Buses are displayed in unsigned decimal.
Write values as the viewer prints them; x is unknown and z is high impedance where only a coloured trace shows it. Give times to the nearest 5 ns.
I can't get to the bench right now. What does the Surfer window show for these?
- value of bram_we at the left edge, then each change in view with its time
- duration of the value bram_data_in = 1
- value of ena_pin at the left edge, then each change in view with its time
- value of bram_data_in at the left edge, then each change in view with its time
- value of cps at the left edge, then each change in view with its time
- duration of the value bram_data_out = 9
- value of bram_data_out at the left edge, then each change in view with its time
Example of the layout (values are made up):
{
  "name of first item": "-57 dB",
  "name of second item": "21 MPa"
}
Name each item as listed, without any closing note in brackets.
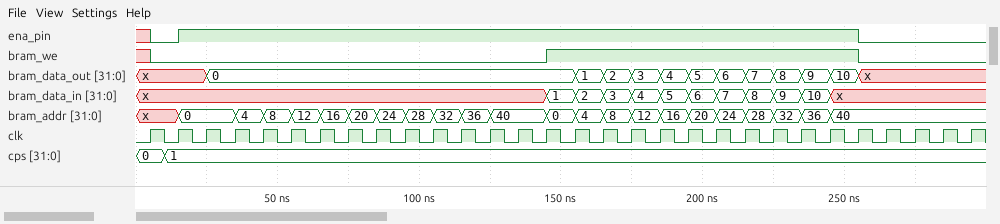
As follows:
{
  "value of bram_we at the left edge, then each change in view with its time": "x, 0 at 5 ns, 1 at 145 ns, 0 at 255 ns",
  "duration of the value bram_data_in = 1": "10 ns",
  "value of ena_pin at the left edge, then each change in view with its time": "x, 0 at 5 ns, 1 at 15 ns, 0 at 255 ns",
  "value of bram_data_in at the left edge, then each change in view with its time": "x, 1 at 145 ns, 2 at 155 ns, 3 at 165 ns, 4 at 175 ns, 5 at 185 ns, 6 at 195 ns, 7 at 205 ns, 8 at 215 ns, 9 at 225 ns, 10 at 235 ns, x at 245 ns",
  "value of cps at the left edge, then each change in view with its time": "0, 1 at 10 ns",
  "duration of the value bram_data_out = 9": "10 ns",
  "value of bram_data_out at the left edge, then each change in view with its time": "x, 0 at 25 ns, 1 at 155 ns, 2 at 165 ns, 3 at 175 ns, 4 at 185 ns, 5 at 195 ns, 6 at 205 ns, 7 at 215 ns, 8 at 225 ns, 9 at 235 ns, 10 at 245 ns, x at 255 ns"
}
